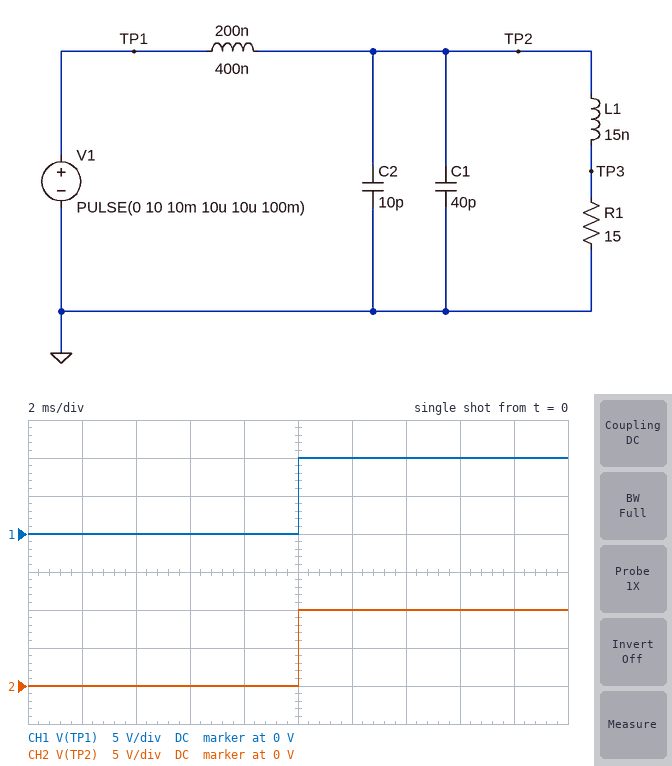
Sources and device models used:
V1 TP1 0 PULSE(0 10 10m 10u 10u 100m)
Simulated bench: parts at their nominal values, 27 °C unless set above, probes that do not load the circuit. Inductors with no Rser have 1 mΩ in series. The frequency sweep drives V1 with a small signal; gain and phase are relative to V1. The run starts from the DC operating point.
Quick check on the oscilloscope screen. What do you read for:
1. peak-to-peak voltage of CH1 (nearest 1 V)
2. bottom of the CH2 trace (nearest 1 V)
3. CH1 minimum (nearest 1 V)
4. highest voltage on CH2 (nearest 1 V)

10 V
0 V
0 V
10 V
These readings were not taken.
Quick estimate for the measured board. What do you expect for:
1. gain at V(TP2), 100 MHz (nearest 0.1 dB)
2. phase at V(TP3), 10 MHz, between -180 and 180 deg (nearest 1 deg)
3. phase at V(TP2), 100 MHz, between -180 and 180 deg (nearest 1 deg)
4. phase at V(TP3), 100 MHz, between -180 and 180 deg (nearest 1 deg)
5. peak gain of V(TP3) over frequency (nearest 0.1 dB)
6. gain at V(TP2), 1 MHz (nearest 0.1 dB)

-21.6 dB
-62 deg
-87 deg
-119 deg
0 dB
-0.1 dB
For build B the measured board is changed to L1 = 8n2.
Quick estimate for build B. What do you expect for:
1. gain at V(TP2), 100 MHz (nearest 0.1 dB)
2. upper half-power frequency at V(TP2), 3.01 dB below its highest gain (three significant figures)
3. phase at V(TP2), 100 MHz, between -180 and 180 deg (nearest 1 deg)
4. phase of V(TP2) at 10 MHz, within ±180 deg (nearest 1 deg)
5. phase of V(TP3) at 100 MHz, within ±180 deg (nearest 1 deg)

-23.6 dB
6.02 MHz
-97 deg
-60 deg
-116 deg
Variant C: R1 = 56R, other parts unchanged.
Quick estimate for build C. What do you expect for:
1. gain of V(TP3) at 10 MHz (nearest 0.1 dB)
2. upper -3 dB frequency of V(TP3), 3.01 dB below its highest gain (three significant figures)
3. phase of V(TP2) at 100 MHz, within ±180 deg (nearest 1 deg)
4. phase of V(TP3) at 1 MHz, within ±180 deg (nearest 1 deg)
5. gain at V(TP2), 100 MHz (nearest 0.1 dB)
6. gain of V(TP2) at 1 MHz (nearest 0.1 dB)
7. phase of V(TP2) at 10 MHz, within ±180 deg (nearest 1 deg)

-0.3 dB
30.7 MHz
-145 deg
-3 deg
-17.6 dB
0 dB
-26 deg
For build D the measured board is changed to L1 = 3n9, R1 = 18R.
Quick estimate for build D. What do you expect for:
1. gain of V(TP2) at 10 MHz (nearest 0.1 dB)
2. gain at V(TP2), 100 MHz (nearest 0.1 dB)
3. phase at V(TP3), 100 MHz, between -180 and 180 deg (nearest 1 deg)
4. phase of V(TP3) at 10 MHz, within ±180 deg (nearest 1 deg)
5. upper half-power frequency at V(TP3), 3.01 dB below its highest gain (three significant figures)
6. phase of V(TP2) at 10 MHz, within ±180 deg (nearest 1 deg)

-4.5 dB
-23.3 dB
-118 deg
-57 deg
7.39 MHz
-56 deg
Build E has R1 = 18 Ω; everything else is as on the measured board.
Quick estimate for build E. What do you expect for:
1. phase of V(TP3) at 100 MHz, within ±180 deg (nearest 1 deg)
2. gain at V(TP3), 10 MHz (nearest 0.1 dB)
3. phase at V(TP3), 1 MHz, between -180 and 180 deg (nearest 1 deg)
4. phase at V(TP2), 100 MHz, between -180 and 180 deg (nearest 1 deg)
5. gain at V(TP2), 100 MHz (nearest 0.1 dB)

-124 deg
-4.7 dB
-8 deg
-96 deg
-20.8 dB
